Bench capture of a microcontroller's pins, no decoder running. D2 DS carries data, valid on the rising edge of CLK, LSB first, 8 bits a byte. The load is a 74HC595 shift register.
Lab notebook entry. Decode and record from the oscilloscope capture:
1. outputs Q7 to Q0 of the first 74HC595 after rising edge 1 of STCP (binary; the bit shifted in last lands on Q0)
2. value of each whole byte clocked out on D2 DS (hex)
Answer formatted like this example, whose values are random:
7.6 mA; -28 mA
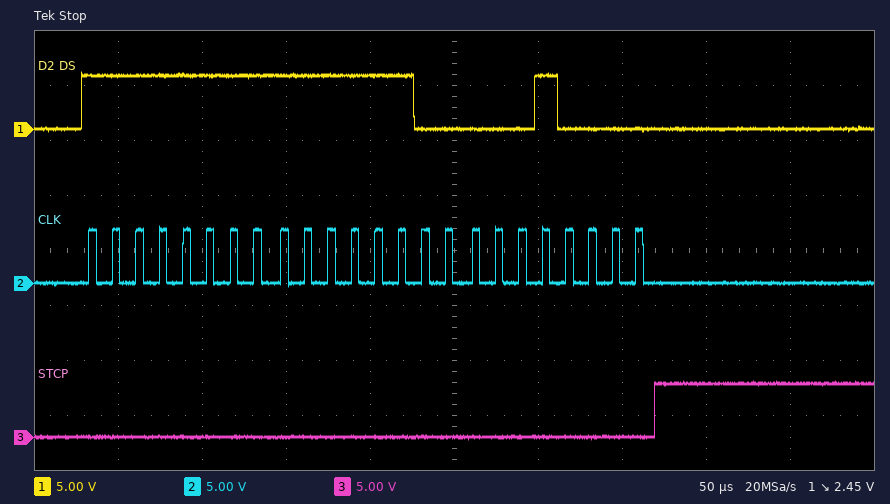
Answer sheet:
00010000; FF 3F 08
